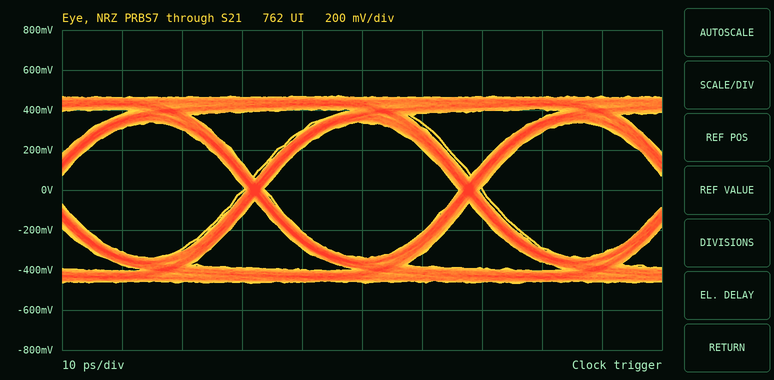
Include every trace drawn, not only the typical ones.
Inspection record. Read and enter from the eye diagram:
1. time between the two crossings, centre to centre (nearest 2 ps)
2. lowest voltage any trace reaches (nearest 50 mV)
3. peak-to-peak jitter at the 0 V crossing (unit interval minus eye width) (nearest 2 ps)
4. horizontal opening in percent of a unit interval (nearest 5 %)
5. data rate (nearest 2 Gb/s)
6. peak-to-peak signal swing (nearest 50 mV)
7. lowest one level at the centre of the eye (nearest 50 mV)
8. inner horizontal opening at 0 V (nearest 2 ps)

36 ps
-450 mV
4 ps
90 %
28 Gb/s
950 mV
350 mV
32 ps
